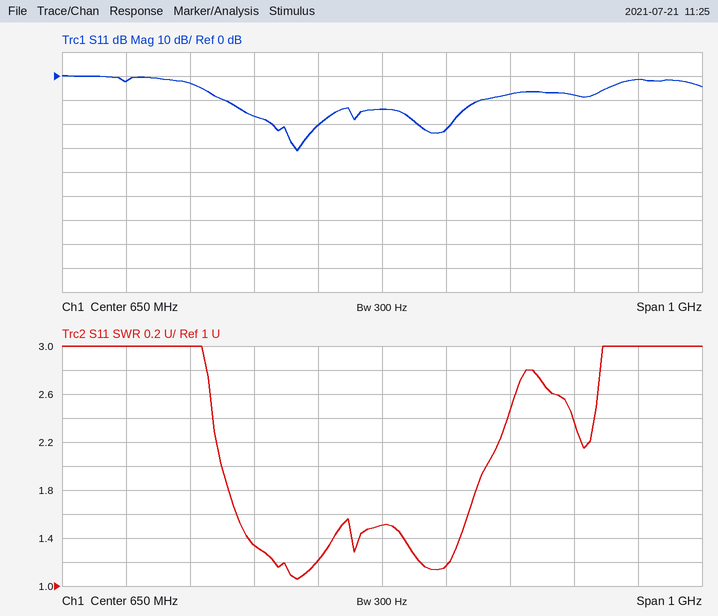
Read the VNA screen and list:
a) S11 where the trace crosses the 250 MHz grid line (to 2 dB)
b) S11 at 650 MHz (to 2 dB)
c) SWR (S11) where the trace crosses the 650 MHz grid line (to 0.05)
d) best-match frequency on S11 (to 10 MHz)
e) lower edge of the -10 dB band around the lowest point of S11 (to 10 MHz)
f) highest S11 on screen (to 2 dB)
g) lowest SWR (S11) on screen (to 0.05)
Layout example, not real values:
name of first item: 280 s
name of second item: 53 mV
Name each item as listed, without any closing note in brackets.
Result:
S11 where the trace crosses the 250 MHz grid line: -2 dB
S11 at 650 MHz: -14 dB
SWR (S11) where the trace crosses the 650 MHz grid line: 1.50
best-match frequency on S11: 520 MHz
lower edge of the -10 dB band around the lowest point of S11: 400 MHz
highest S11 on screen: 0 dB
lowest SWR (S11) on screen: 1.05
